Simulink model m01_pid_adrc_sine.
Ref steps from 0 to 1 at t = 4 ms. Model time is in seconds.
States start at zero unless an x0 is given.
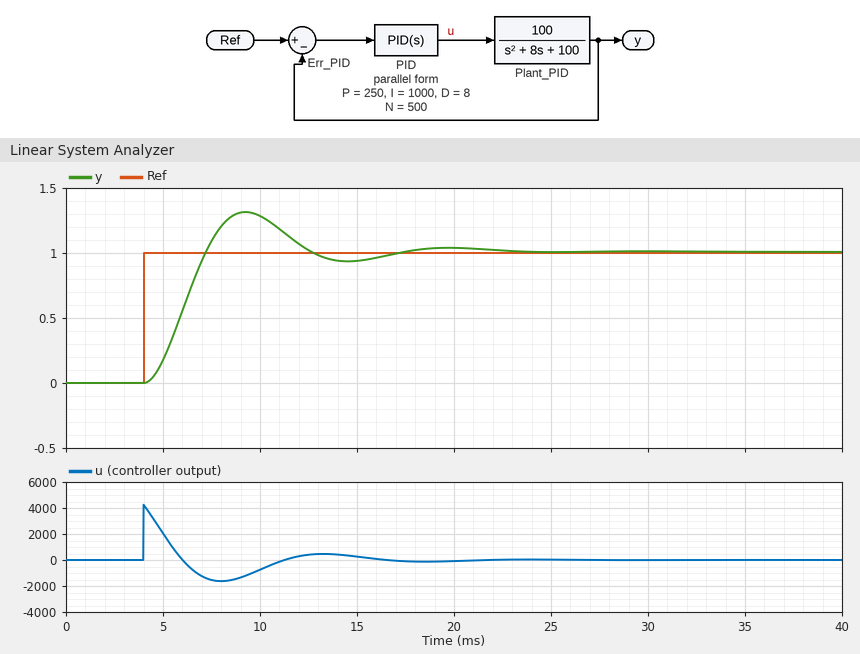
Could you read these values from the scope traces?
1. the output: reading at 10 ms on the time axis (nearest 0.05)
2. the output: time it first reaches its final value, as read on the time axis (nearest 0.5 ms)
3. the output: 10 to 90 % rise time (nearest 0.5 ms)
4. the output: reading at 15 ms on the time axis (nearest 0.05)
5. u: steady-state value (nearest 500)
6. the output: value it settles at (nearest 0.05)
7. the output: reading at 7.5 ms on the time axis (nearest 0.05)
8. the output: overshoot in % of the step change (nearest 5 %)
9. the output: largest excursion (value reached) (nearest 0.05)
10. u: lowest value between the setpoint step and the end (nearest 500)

1.30
7.0 ms
2.0 ms
0.95
0
1.00
1.10
30 %
1.30
-1500
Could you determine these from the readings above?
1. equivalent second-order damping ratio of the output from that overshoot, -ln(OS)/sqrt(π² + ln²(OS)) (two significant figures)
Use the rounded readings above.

0.36
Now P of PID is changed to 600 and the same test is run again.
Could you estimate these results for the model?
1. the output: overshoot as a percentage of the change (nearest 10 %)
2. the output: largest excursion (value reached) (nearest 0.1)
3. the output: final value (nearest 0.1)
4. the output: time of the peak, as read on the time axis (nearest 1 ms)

40 %
1.4
1.0
9 ms
